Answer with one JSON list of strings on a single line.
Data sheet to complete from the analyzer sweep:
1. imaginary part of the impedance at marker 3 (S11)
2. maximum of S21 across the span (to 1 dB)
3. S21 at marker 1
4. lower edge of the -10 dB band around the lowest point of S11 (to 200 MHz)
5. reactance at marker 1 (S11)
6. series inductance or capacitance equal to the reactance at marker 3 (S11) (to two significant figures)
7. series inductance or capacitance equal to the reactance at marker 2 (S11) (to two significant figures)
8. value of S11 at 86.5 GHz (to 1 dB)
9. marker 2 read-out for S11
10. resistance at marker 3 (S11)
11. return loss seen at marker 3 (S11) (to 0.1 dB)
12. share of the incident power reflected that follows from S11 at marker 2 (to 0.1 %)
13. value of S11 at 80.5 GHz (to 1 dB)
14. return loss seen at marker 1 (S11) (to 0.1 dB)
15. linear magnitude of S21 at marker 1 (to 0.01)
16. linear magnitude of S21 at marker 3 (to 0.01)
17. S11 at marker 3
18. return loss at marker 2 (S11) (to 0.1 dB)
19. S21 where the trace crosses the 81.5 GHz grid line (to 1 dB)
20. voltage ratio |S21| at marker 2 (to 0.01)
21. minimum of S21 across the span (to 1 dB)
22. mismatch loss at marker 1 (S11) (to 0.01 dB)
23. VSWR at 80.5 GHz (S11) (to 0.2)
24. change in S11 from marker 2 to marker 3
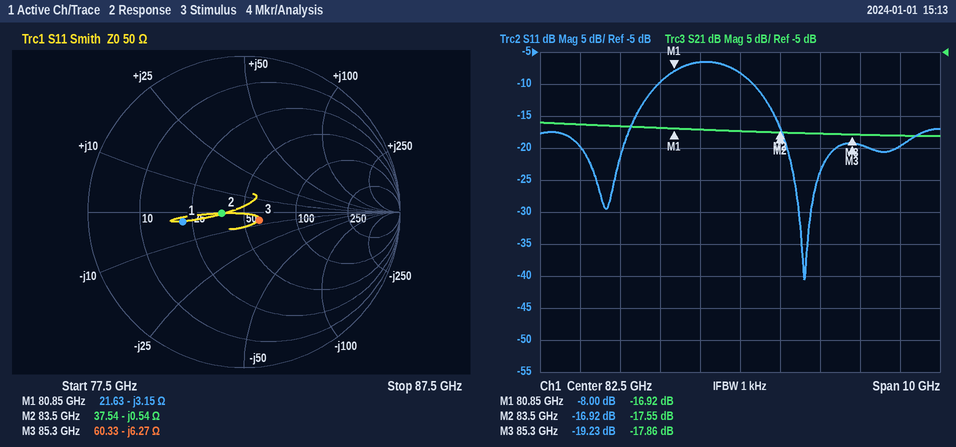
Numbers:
["-6.27 Ω", "-16 dB", "-16.92 dB", "82.8 GHz", "-3.15 Ω", "300 fF", "3.5 pF", "-20 dB", "-16.92 dB", "60.33 Ω", "19.2 dB", "2.0 %", "-10 dB", "8.0 dB", "0.14", "0.13", "-19.23 dB", "16.9 dB", "-17 dB", "0.13", "-18 dB", "0.75 dB", "2.0", "-2.31 dB"]
